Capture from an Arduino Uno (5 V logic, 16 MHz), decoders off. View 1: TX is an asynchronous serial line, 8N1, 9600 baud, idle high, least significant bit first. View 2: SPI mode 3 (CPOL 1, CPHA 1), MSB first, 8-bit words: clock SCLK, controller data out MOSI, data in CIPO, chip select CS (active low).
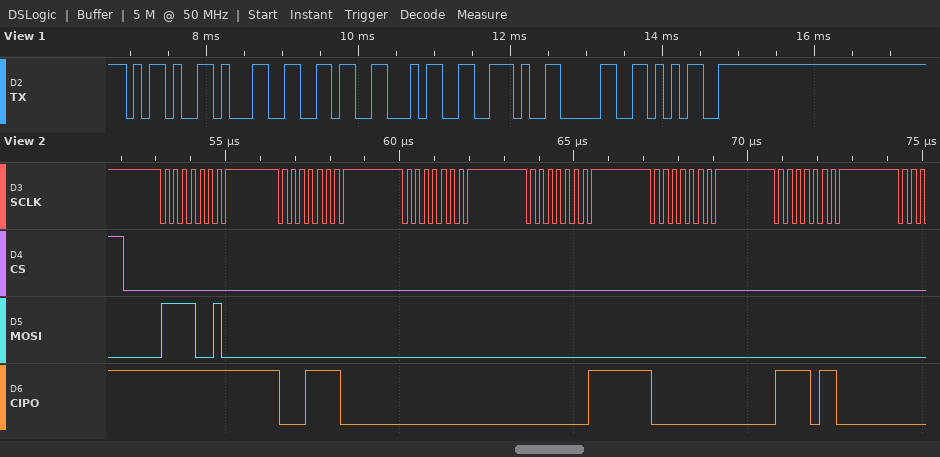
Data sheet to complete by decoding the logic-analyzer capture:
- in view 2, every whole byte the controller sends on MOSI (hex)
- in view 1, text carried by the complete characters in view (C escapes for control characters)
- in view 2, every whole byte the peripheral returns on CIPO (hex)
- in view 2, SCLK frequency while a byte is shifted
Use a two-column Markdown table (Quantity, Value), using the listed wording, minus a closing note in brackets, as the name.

| Quantity | Value |
|---|---|
| in view 2, every whole byte the controller sends on MOSI | F2 00 00 00 00 00 |
| in view 1, text carried by the complete characters in view | "-164.05" |
| in view 2, every whole byte the peripheral returns on CIPO | FF 1E 00 01 00 F6 |
| in view 2, SCLK frequency while a byte is shifted | 4 MHz |
